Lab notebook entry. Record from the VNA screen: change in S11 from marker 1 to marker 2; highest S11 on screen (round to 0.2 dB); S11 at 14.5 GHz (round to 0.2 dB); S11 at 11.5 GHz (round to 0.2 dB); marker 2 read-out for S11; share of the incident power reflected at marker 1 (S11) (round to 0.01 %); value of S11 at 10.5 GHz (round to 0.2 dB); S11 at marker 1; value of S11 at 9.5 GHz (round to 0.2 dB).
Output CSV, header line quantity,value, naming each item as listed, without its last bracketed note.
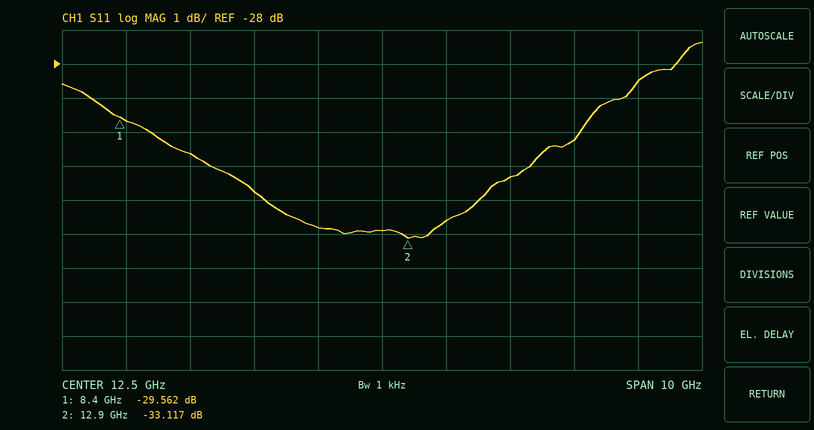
quantity,value
change in S11 from marker 1 to marker 2,-3.555 dB
highest S11 on screen,-27.4 dB
S11 at 14.5 GHz,-31.4 dB
S11 at 11.5 GHz,-32.8 dB
marker 2 read-out for S11,-33.117 dB
share of the incident power reflected at marker 1 (S11),0.11 %
value of S11 at 10.5 GHz,-31.8 dB
S11 at marker 1,-29.562 dB
value of S11 at 9.5 GHz,-30.6 dB
